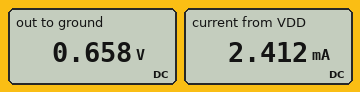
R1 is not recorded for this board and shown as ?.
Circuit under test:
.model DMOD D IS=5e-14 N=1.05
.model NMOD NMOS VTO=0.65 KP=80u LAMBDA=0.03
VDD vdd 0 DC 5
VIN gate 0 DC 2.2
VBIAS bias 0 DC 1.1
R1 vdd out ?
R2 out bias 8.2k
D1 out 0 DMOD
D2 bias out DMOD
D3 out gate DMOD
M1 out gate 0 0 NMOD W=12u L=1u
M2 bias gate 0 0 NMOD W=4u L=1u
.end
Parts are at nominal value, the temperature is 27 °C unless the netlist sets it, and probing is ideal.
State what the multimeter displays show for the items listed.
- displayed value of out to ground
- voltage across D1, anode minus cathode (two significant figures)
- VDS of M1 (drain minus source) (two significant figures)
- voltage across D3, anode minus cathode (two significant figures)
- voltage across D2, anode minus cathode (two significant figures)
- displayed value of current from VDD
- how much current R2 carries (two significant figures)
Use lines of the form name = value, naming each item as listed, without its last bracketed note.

displayed value of out to ground = 0.658 V
voltage across D1, anode minus cathode = 660 mV
VDS of M1 (drain minus source) = 660 mV
voltage across D3, anode minus cathode = -1.5 V
voltage across D2, anode minus cathode = 440 mV
displayed value of current from VDD = 2.412 mA
how much current R2 carries = 54 µA
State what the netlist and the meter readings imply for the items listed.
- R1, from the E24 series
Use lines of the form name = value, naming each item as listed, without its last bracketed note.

R1, from the E24 series = 1.8 kΩ
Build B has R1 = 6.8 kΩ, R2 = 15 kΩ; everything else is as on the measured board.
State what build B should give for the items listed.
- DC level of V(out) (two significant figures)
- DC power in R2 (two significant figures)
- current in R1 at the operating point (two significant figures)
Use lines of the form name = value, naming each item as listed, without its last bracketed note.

DC level of V(out) = 550 mV
DC power in R2 = 20 µW
current in R1 at the operating point = 650 µA
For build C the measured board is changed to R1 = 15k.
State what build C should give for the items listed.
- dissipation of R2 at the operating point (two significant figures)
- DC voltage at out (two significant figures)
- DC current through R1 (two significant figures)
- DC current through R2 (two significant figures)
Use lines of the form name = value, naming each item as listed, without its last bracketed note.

dissipation of R2 at the operating point = 45 µW
DC voltage at out = 490 mV
DC current through R1 = 300 µA
DC current through R2 = 74 µA
